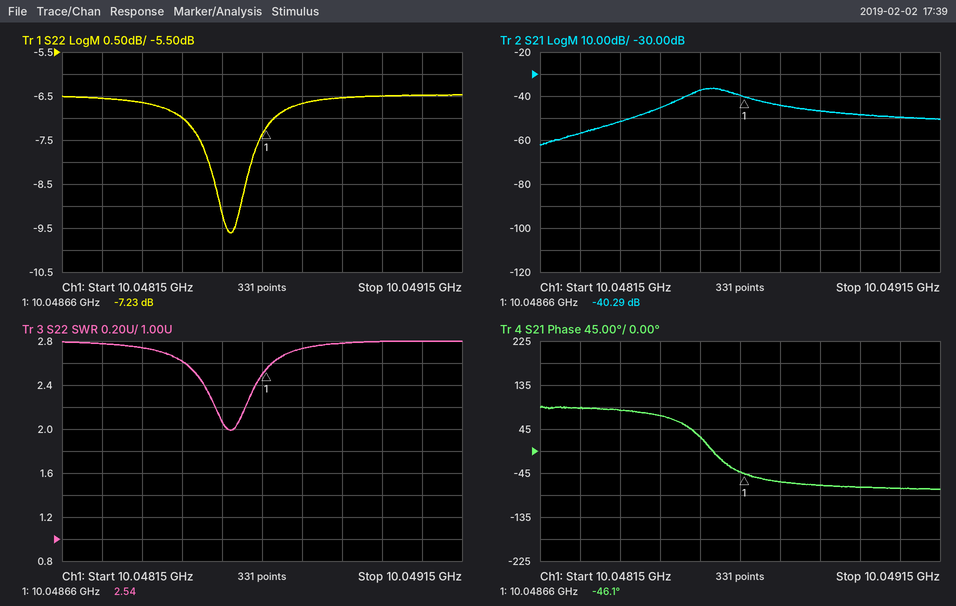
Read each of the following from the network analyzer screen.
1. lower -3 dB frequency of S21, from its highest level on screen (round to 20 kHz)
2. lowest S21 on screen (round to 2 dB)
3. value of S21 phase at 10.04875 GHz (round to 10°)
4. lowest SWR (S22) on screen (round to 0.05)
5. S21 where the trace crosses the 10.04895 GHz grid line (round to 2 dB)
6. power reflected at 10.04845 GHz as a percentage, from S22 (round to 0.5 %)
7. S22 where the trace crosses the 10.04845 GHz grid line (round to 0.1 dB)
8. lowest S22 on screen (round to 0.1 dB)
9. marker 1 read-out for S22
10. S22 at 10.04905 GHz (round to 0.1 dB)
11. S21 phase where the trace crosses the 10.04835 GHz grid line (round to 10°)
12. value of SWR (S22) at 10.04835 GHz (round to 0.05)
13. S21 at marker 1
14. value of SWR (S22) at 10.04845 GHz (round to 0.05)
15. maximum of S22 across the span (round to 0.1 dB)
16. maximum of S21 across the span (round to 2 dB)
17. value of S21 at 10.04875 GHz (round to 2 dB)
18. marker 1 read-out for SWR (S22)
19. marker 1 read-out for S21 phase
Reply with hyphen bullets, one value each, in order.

- 10.04852 GHz
- -62 dB
- -60°
- 2.00
- -48 dB
- 20.0 %
- -7.0 dB
- -9.6 dB
- -7.23 dB
- -6.5 dB
- 80°
- 2.75
- -40.29 dB
- 2.60
- -6.5 dB
- -36 dB
- -44 dB
- 2.54
- -46.1°
